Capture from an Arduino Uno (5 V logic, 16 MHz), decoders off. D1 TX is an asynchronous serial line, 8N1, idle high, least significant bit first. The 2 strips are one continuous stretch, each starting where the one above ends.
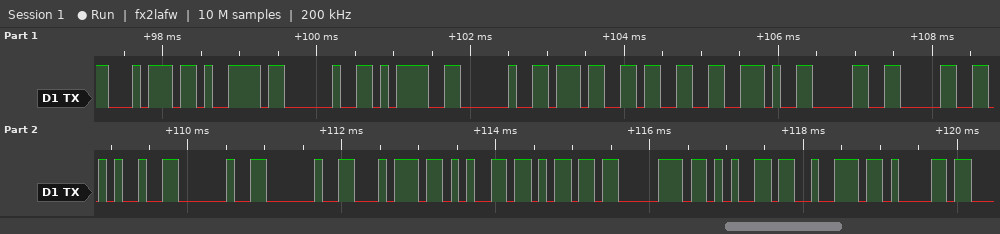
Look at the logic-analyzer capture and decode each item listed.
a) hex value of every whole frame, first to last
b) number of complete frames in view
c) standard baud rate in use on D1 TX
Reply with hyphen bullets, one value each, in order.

- 0x74 0x79 0x20 0x3D 0x20 0x37 0x33 0x2E 0x30 0x30 0x25 0x20 0x20 0x74 0x65 0x6D 0x70 0x65 0x72 0x61
- 20
- 9600 baud
